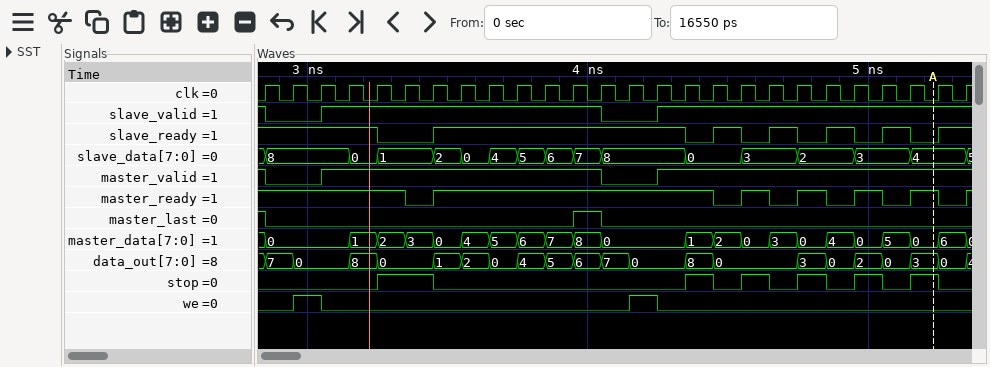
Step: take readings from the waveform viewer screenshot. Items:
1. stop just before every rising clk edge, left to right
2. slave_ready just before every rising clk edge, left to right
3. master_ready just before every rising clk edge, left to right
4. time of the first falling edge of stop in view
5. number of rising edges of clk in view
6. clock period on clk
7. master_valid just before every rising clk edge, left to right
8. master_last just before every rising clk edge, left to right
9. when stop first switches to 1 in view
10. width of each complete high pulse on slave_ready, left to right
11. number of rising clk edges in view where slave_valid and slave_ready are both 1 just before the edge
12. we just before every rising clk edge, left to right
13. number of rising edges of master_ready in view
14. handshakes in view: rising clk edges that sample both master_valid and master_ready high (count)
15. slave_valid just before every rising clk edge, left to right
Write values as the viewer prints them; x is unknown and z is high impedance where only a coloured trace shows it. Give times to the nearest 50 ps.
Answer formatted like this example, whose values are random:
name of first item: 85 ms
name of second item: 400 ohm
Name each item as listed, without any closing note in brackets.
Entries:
stop just before every rising clk edge, left to right: 0 0 0 0 0 1 1 0 0 0 0 0 0 0 0 0 1 0 1 0 1 0 1 0 1 0
slave_ready just before every rising clk edge, left to right: 1 1 1 1 1 0 0 1 1 1 1 1 1 1 1 1 0 1 0 1 0 1 0 1 0 1
master_ready just before every rising clk edge, left to right: 1 1 1 1 1 1 0 1 1 1 1 1 1 1 1 1 1 0 1 0 1 0 1 0 1 0
time of the first falling edge of stop in view: 3450 ps
number of rising edges of clk in view: 26
clock period on clk: 100 ps
master_valid just before every rising clk edge, left to right: 1 0 0 1 1 1 1 1 1 1 1 1 1 0 0 1 1 1 1 1 1 1 1 1 1 1
master_last just before every rising clk edge, left to right: 1 0 0 0 0 0 0 0 0 0 0 0 1 0 0 0 0 0 0 0 0 0 0 0 0 0
when stop first switches to 1 in view: 3250 ps
width of each complete high pulse on slave_ready, left to right: 900 ps, 100 ps, 100 ps, 100 ps, 100 ps
number of rising clk edges in view where slave_valid and slave_ready are both 1 just before the edge: 15
we just before every rising clk edge, left to right: 0 0 1 0 0 0 0 0 0 0 0 0 0 0 1 0 0 0 0 0 0 0 0 0 0 0
number of rising edges of master_ready in view: 6
handshakes in view: rising clk edges that sample both master_valid and master_ready high: 16
slave_valid just before every rising clk edge, left to right: 1 0 0 1 1 1 1 1 1 1 1 1 1 0 0 1 1 1 1 1 1 1 1 1 1 1
